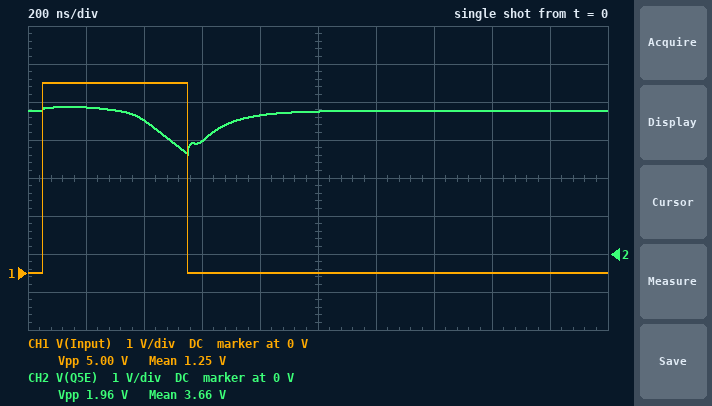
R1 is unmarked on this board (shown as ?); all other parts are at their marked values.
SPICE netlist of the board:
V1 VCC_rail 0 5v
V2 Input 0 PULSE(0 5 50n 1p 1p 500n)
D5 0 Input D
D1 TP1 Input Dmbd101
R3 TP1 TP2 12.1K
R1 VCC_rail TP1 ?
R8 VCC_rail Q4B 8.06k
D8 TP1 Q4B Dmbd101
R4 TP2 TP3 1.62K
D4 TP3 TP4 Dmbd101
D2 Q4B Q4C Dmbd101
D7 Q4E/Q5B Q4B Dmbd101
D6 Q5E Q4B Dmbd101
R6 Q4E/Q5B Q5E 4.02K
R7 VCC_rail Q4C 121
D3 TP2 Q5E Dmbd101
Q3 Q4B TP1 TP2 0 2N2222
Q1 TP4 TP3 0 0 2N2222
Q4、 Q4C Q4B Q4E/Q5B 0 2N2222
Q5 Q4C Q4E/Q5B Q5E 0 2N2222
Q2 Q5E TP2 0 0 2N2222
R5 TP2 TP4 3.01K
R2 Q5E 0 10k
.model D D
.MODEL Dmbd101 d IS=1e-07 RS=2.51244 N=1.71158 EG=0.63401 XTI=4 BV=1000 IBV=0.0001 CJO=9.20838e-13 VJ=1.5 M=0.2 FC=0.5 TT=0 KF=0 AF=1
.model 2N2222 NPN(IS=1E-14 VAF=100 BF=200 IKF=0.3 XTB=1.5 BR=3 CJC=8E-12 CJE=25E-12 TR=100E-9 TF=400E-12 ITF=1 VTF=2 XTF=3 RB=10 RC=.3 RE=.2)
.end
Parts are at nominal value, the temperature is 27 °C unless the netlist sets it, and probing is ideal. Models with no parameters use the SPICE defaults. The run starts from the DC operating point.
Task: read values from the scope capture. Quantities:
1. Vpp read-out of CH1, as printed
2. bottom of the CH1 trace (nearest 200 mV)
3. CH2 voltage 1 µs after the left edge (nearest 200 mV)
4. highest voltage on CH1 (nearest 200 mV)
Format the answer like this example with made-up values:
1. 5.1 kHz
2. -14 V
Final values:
1. 5.00 V
2. 0 V
3. 3.8 V
4. 5.0 V
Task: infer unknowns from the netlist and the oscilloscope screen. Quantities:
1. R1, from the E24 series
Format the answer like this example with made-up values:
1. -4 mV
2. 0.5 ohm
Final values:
1. 43 kΩ
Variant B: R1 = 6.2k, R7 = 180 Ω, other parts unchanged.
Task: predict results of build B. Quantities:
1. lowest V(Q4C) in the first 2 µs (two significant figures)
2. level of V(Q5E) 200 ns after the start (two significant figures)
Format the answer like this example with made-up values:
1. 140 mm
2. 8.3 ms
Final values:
1. 1.9 V
2. 250 mV
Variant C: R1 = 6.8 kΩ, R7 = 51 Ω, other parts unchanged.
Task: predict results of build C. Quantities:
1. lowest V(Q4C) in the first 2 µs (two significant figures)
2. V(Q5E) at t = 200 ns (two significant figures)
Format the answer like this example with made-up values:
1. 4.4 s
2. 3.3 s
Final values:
1. 3.3 V
2. 250 mV
